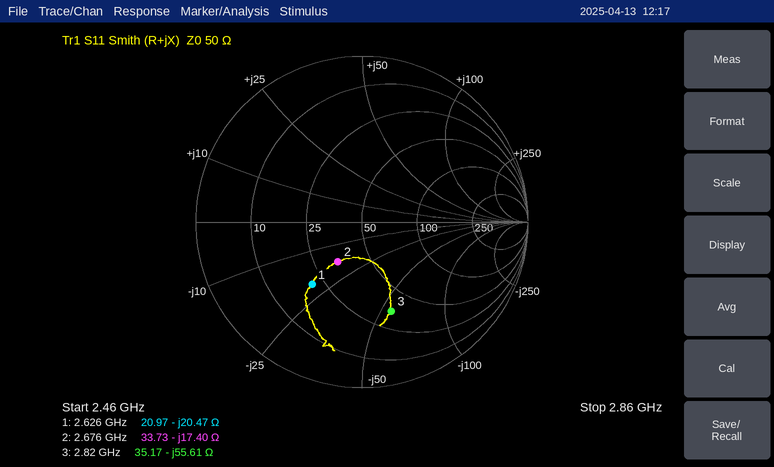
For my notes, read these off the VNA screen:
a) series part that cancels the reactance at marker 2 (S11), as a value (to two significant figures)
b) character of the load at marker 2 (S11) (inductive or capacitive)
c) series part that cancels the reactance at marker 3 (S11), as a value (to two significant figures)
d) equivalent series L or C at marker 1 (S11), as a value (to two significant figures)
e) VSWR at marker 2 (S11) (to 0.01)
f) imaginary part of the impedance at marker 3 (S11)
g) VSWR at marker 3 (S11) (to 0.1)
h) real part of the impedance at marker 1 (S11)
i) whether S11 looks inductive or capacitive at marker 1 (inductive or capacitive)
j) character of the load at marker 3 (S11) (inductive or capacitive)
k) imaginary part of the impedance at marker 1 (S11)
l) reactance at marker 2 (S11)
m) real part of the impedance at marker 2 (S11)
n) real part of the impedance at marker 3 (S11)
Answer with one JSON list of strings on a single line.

["1.0 nH", "capacitive", "3.1 nH", "3.0 pF", "1.77", "-55.61 Ω", "3.6", "20.97 Ω", "capacitive", "capacitive", "-20.47 Ω", "-17.40 Ω", "33.73 Ω", "35.17 Ω"]
